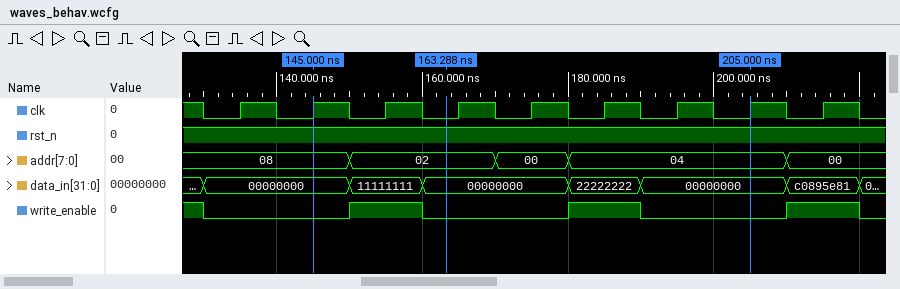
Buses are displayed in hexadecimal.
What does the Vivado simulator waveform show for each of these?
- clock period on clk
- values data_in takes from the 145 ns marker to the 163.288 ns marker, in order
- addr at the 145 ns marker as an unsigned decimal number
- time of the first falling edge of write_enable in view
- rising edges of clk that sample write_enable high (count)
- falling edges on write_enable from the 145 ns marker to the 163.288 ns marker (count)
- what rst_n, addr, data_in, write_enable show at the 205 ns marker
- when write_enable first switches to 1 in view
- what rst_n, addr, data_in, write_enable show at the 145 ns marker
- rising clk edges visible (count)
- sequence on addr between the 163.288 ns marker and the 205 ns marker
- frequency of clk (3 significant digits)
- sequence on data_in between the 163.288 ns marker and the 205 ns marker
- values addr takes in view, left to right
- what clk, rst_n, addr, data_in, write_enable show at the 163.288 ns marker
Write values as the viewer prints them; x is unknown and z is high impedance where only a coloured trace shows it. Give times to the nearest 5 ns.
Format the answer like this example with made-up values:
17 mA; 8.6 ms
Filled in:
10 ns; 00000000, 11111111, 00000000; 8; 130 ns; 3; 1; rst_n=1, addr=04, data_in=00000000, write_enable=0; 150 ns; rst_n=1, addr=08, data_in=00000000, write_enable=0; 9; 02, 00, 04; 100 MHz; 00000000, 22222222, 00000000; 08, 02, 00, 04, 00; clk=0, rst_n=1, addr=02, data_in=00000000, write_enable=0
